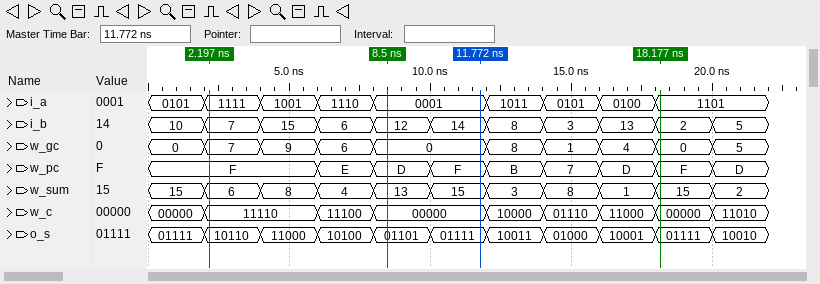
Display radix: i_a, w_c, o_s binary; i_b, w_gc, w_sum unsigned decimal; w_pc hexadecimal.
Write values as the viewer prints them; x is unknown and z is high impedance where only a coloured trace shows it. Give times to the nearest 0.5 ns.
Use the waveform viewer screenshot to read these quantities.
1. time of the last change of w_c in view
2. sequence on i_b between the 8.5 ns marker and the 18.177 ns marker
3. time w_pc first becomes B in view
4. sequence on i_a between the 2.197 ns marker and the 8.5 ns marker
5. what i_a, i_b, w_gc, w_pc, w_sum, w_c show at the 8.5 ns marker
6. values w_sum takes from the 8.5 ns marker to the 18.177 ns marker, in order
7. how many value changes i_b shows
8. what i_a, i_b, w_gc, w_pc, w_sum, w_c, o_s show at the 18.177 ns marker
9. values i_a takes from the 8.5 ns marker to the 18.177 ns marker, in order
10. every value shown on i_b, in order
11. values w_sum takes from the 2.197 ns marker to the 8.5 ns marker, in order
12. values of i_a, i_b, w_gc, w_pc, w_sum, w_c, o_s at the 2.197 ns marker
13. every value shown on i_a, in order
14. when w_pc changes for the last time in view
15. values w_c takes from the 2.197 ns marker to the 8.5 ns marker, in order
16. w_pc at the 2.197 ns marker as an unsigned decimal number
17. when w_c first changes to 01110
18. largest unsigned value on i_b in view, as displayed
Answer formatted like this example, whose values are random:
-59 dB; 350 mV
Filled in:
20 ns; 12, 14, 8, 3, 13, 2; 12 ns; 1111, 1001, 1110, 0001; i_a=0001, i_b=12, w_gc=0, w_pc=D, w_sum=13, w_c=00000; 13, 15, 3, 8, 1, 15; 10; i_a=1101, i_b=2, w_gc=0, w_pc=F, w_sum=15, w_c=00000, o_s=01111; 0001, 1011, 0101, 0100, 1101; 10, 7, 15, 6, 12, 14, 8, 3, 13, 2, 5; 6, 8, 4, 13; i_a=1111, i_b=7, w_gc=7, w_pc=F, w_sum=6, w_c=11110, o_s=10110; 0101, 1111, 1001, 1110, 0001, 1011, 0101, 0100, 1101; 20 ns; 11110, 11100, 00000; 15; 14 ns; 15
